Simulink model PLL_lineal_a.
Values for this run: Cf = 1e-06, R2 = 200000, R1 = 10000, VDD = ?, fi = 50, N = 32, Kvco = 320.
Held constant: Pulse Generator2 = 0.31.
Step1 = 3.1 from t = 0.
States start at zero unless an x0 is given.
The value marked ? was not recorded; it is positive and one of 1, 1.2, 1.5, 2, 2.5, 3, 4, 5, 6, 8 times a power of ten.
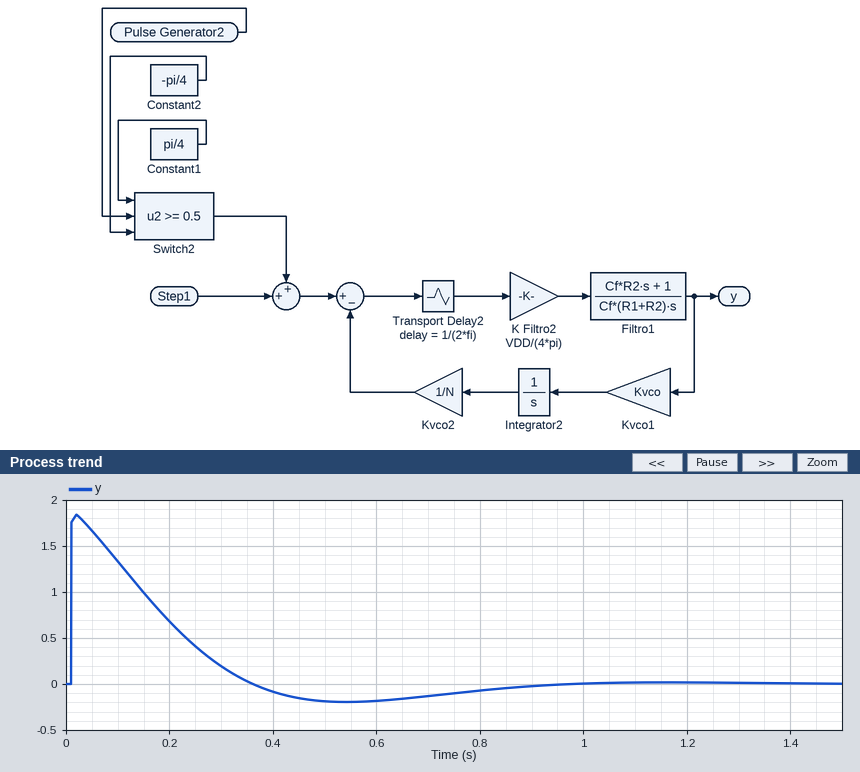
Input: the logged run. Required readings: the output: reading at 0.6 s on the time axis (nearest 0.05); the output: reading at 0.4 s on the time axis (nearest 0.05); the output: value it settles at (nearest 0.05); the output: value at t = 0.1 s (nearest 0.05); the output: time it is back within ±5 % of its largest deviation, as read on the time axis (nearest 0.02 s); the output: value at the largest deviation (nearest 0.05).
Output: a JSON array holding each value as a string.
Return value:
["-0.20", "-0.10", "0.00", "1.35", "0.76 s", "1.85"]
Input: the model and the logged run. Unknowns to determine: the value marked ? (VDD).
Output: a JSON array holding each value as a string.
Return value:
["10"]
